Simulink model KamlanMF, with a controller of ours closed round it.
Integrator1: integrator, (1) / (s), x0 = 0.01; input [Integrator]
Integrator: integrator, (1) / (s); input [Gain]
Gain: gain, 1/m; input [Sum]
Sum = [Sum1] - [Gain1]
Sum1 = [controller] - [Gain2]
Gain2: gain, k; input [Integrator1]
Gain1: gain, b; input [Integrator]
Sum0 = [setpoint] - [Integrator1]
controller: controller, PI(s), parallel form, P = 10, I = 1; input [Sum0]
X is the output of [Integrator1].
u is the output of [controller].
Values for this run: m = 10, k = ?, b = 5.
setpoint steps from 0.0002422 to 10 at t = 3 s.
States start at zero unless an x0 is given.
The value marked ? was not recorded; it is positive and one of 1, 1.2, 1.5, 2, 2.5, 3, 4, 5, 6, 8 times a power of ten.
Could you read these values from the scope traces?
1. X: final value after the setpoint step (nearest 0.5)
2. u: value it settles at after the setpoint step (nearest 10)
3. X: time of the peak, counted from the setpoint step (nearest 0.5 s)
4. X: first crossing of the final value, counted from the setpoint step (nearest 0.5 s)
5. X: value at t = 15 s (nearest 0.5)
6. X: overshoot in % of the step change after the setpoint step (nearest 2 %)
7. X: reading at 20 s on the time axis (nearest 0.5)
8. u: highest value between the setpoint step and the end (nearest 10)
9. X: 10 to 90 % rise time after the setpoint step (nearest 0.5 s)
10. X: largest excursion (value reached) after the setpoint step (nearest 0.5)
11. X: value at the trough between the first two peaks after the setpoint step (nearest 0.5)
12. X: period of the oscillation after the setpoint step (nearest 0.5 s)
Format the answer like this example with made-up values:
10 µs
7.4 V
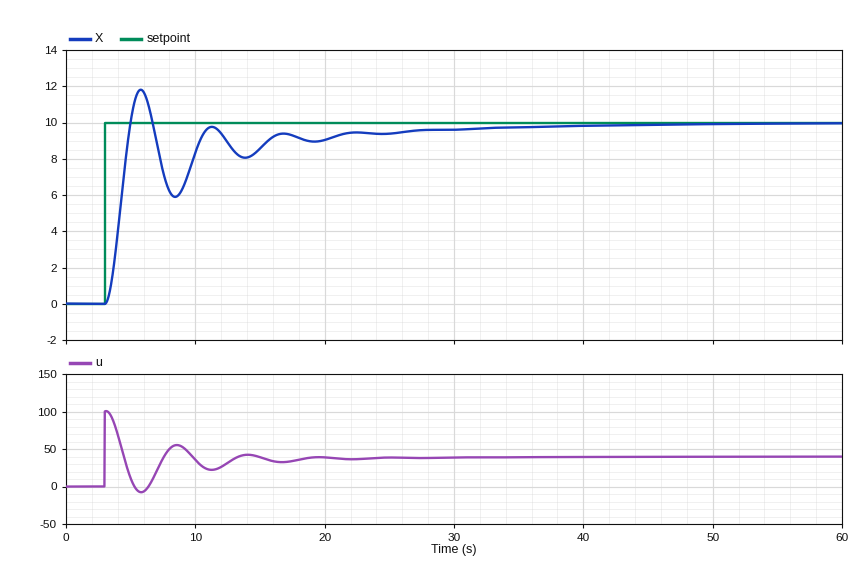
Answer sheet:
10.0
40
3.0 s
2.0 s
8.5
18 %
9.0
100
1.5 s
12.0
6.0
5.5 s
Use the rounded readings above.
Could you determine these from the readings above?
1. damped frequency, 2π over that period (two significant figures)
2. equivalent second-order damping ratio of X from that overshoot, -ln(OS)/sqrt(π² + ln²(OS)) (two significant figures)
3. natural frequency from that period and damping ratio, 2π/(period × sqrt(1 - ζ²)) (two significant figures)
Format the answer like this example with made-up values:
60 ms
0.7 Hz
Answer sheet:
1.1 rad/s
0.48
1.3 rad/s
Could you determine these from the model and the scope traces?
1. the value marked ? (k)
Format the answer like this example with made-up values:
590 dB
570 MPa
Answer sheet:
4
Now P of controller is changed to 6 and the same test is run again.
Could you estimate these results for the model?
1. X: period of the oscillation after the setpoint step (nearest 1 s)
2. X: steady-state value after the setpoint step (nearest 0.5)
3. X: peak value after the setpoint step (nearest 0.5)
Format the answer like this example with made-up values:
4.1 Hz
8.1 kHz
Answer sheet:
7 s
10.0
10.5
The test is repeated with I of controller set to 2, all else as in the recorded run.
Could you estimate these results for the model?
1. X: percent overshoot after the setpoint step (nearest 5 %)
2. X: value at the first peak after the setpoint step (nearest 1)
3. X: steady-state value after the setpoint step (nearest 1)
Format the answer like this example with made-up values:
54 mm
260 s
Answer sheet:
30 %
13
10
